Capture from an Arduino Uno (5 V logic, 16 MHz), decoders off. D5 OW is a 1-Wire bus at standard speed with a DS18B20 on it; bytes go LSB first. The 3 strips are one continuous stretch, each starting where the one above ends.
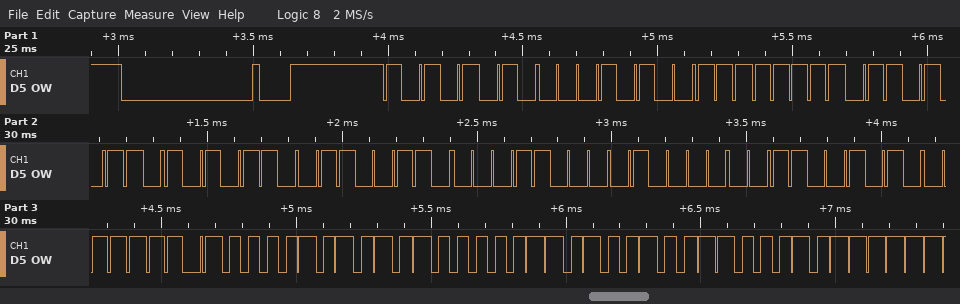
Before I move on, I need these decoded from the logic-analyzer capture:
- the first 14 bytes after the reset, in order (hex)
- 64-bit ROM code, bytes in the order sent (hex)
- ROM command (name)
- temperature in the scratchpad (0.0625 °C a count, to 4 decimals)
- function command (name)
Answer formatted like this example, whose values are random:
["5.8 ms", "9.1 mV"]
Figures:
["55 28 FF D6 6A 66 18 02 53 BE 50 05 4B 46", "28 FF D6 6A 66 18 02 53", "Match ROM", "85.0000 °C", "Read Scratchpad"]
